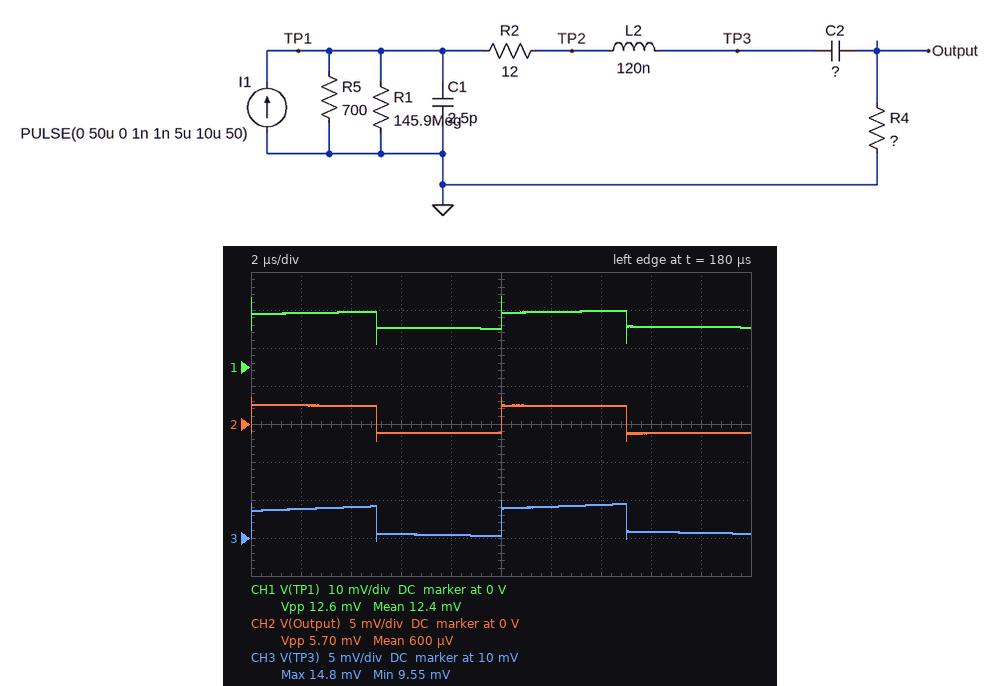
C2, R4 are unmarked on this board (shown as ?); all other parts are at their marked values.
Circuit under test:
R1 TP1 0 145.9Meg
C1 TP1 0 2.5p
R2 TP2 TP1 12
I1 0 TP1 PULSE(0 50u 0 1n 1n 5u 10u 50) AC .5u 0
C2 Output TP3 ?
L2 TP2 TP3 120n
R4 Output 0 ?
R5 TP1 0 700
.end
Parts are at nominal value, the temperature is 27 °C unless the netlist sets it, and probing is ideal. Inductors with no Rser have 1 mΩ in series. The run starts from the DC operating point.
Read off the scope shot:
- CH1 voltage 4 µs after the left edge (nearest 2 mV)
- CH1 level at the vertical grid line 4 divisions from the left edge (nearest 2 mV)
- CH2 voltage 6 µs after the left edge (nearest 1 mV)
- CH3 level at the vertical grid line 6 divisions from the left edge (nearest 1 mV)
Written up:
14 mV
10 mV
-1 mV
14 mV
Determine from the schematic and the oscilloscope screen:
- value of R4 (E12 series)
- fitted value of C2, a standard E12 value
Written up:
82 Ω
220 nF
